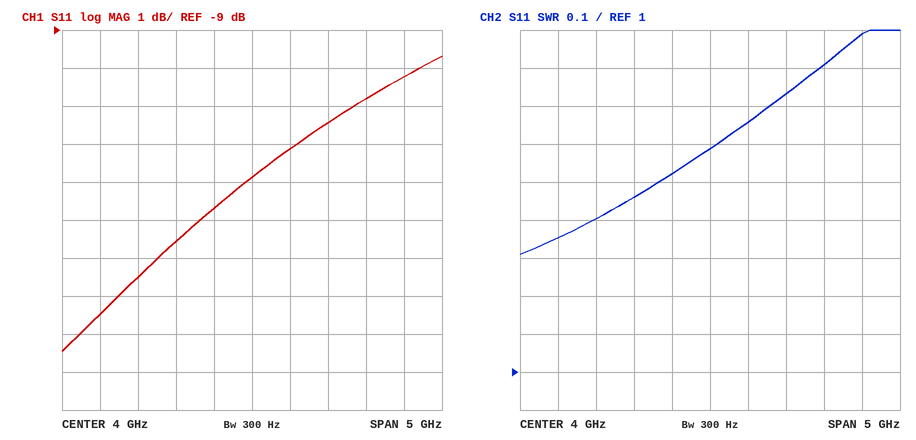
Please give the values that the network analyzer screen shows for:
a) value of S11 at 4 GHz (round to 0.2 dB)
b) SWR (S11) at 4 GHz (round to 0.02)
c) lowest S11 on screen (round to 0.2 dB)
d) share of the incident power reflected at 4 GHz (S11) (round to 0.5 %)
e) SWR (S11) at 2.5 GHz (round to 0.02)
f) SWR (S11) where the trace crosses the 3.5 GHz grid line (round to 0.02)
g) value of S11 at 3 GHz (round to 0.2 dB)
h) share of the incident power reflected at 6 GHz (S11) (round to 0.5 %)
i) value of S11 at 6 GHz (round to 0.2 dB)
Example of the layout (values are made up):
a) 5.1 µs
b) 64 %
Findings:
a) -12.8 dB
b) 1.58
c) -17.4 dB
d) 5.0 %
e) 1.40
f) 1.52
g) -14.6 dB
h) 9.5 %
i) -10.2 dB
